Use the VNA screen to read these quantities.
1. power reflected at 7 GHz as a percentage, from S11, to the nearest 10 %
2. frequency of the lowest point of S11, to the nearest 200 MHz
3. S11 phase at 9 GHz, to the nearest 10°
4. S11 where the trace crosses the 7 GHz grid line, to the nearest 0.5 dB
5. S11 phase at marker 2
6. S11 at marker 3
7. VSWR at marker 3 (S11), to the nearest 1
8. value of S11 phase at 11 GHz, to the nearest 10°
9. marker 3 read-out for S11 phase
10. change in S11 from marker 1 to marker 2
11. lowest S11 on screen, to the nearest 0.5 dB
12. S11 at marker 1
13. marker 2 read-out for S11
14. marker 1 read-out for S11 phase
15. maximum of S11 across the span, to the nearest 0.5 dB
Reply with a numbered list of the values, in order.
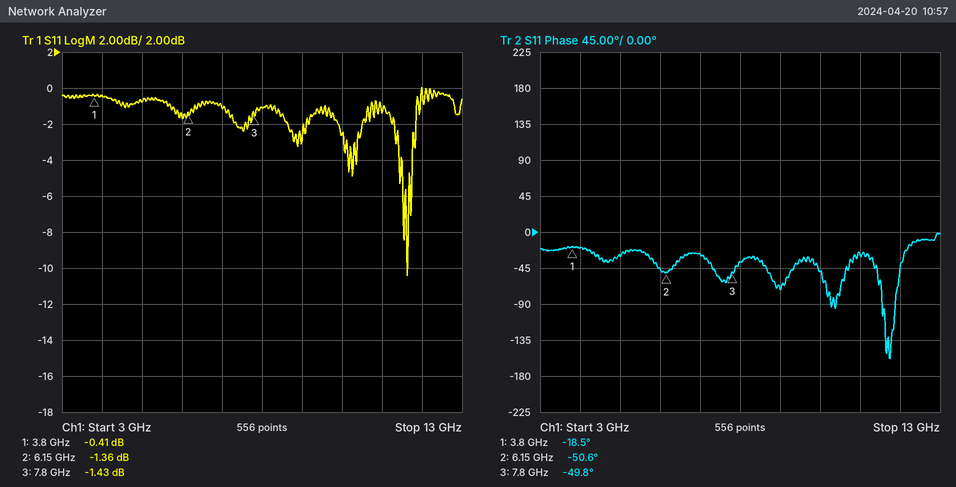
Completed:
1. 80 %
2. 11.6 GHz
3. -70°
4. -1.0 dB
5. -50.6°
6. -1.43 dB
7. 12
8. -30°
9. -49.8°
10. -0.95 dB
11. -10.5 dB
12. -0.41 dB
13. -1.36 dB
14. -18.5°
15. 0.0 dB
